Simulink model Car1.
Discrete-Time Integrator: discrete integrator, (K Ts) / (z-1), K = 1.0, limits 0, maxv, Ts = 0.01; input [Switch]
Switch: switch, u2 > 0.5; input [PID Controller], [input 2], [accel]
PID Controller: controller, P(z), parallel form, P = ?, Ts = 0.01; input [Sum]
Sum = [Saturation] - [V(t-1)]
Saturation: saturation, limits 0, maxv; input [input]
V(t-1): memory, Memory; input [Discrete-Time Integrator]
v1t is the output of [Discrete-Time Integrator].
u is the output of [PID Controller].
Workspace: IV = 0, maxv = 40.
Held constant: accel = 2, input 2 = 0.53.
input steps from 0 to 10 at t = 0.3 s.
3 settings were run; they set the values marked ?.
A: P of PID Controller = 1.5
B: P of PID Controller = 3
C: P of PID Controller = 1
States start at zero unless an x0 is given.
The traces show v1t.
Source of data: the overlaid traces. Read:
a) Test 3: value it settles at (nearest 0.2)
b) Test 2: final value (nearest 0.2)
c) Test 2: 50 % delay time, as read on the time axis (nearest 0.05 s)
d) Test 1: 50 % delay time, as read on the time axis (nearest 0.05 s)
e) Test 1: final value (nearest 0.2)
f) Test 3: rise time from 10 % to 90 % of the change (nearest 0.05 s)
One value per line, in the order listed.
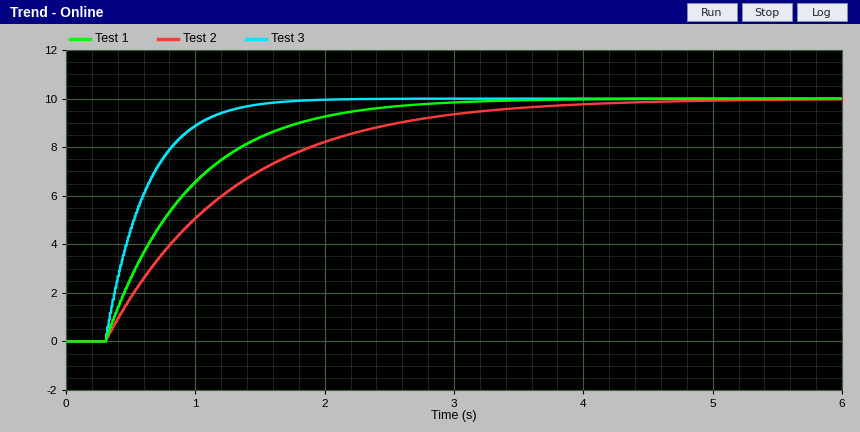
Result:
10.0
10.0
1.00 s
0.75 s
10.0
0.70 s
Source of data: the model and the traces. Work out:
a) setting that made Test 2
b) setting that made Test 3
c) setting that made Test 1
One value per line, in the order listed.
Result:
C
B
A
